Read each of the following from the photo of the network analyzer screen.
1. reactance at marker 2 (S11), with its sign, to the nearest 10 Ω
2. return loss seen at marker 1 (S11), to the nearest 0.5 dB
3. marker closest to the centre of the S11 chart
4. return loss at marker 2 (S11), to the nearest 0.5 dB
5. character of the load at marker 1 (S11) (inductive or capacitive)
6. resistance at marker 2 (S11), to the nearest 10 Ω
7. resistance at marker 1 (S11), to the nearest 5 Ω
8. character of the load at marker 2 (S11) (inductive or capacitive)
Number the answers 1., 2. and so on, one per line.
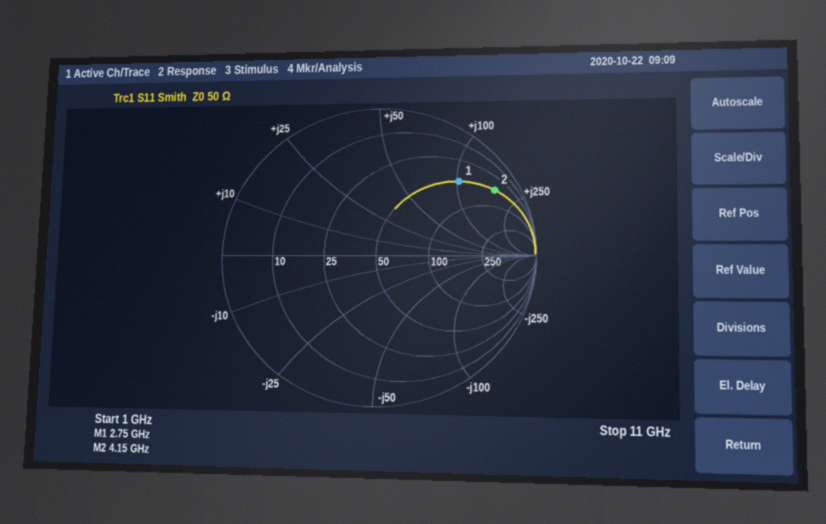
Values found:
1. +170 Ω
2. 3.0 dB
3. marker 1
4. 1.5 dB
5. inductive
6. 50 Ω
7. 50 Ω
8. inductive
